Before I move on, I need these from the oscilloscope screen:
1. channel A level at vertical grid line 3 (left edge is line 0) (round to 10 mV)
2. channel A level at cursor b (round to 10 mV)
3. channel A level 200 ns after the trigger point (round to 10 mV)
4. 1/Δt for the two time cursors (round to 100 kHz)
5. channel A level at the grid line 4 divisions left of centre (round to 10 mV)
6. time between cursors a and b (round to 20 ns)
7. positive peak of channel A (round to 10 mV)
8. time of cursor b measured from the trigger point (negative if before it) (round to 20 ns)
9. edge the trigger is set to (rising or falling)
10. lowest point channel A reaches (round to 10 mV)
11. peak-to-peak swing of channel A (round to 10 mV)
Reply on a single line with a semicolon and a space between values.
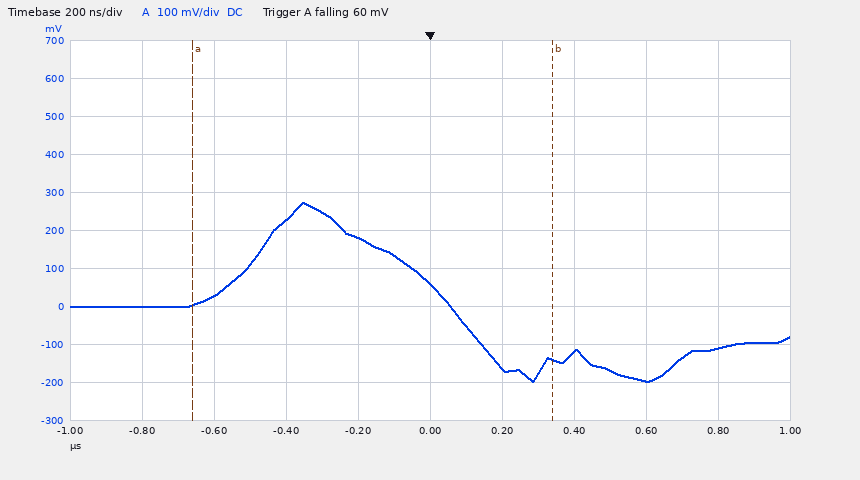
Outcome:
230 mV; -140 mV; -160 mV; 1.0 MHz; 0 mV; 1.00 µs; 270 mV; +340 ns; falling; -200 mV; 470 mV
